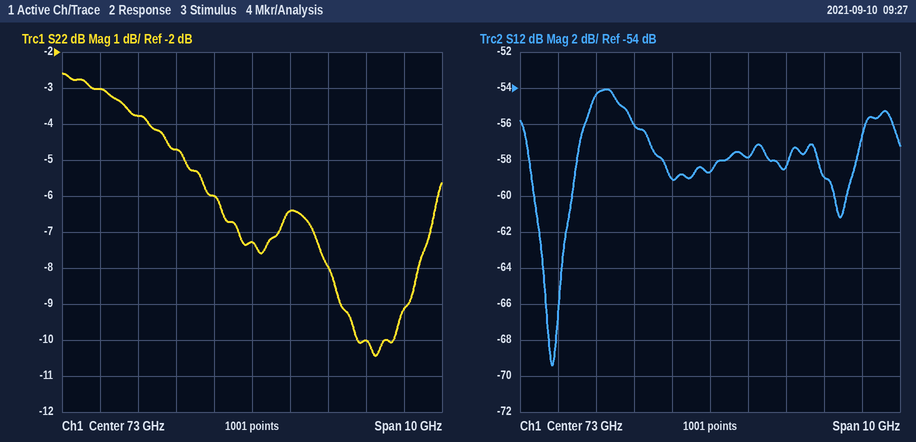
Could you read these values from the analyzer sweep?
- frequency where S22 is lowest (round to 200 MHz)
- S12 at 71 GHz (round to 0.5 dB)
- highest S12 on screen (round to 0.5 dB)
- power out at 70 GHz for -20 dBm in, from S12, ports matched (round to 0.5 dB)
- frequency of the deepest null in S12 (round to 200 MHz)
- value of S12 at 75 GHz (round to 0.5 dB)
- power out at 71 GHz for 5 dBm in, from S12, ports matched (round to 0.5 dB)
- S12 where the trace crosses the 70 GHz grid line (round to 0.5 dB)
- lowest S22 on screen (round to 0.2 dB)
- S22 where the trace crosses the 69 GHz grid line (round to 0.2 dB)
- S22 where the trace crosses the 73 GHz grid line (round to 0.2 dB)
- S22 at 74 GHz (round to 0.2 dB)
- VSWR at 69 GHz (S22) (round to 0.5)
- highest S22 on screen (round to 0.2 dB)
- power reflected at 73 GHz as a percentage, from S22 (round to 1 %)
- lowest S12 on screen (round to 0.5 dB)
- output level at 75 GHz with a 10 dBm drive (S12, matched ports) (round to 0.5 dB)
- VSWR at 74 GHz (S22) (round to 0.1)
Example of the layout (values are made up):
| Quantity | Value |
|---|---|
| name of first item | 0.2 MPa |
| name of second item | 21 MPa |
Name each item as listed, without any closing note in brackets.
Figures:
| Quantity | Value |
|---|---|
| frequency where S22 is lowest | 76.2 GHz |
| S12 at 71 GHz | -56.0 dB |
| highest S12 on screen | -54.0 dB |
| power out at 70 GHz for -20 dBm in, from S12, ports matched | -74.5 dBm |
| frequency of the deepest null in S12 | 68.8 GHz |
| value of S12 at 75 GHz | -58.5 dB |
| power out at 71 GHz for 5 dBm in, from S12, ports matched | -51.0 dBm |
| S12 where the trace crosses the 70 GHz grid line | -54.5 dB |
| lowest S22 on screen | -10.4 dB |
| S22 where the trace crosses the 69 GHz grid line | -3.0 dB |
| S22 where the trace crosses the 73 GHz grid line | -7.2 dB |
| S22 at 74 GHz | -6.4 dB |
| VSWR at 69 GHz (S22) | 6.0 |
| highest S22 on screen | -2.6 dB |
| power reflected at 73 GHz as a percentage, from S22 | 19 % |
| lowest S12 on screen | -69.5 dB |
| output level at 75 GHz with a 10 dBm drive (S12, matched ports) | -48.5 dBm |
| VSWR at 74 GHz (S22) | 2.8 |
